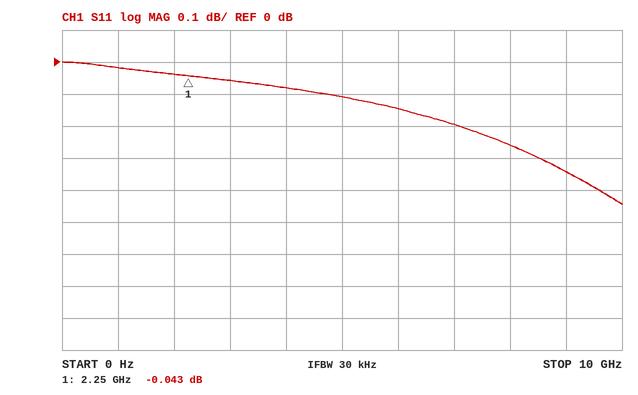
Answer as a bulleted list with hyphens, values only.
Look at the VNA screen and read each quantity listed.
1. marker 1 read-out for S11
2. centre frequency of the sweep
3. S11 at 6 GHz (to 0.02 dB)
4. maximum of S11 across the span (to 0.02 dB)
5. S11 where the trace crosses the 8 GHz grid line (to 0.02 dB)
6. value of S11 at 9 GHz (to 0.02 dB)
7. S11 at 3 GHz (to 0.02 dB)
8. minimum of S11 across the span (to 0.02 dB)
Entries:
- -0.043 dB
- 5 GHz
- -0.14 dB
- 0.00 dB
- -0.26 dB
- -0.34 dB
- -0.06 dB
- -0.44 dB
